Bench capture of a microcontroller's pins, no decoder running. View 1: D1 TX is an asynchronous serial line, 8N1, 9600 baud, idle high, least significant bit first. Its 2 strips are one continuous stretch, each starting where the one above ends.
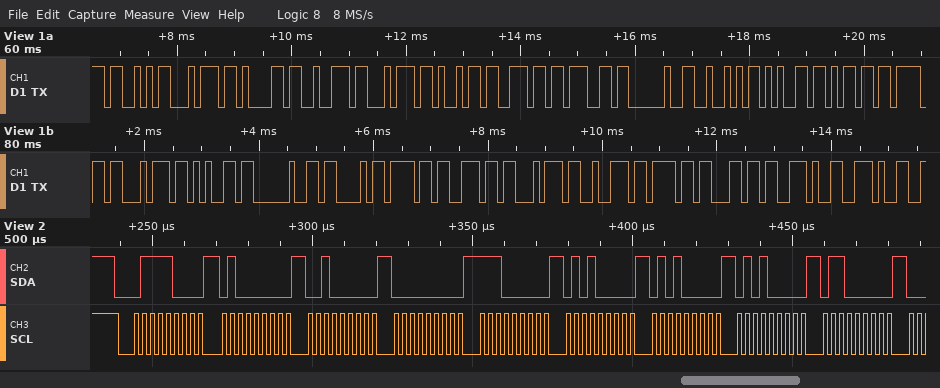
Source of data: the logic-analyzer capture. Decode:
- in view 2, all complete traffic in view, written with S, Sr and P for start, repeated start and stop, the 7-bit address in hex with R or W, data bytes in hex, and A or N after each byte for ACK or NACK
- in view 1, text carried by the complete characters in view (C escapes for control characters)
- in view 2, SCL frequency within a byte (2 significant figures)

S 3CW A 40 A 20 A 00 A E0 A 50 A 50 A 50 A 60 A
"Starting Remote Control.."
400 kHz
